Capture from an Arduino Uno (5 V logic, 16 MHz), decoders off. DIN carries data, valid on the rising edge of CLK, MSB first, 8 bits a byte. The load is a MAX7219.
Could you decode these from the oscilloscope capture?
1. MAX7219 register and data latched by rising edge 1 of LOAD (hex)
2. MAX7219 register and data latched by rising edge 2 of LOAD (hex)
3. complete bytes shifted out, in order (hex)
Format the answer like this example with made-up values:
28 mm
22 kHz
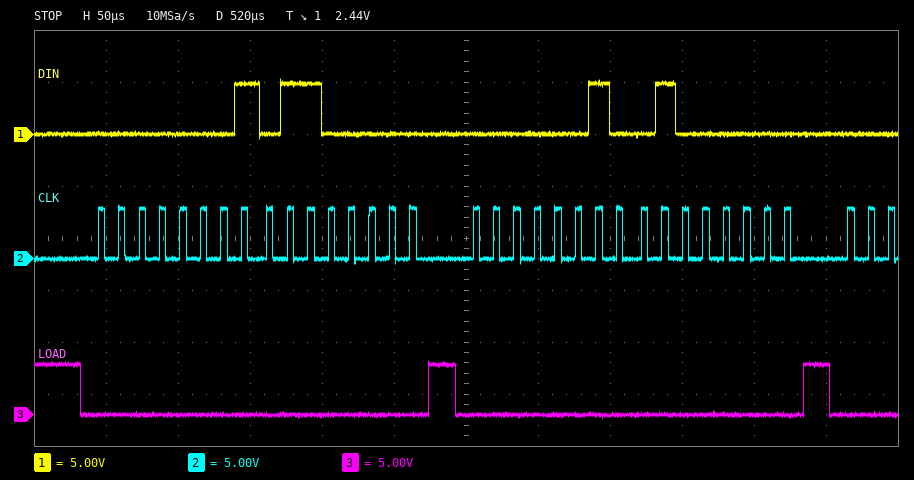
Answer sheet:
register 0x1, data 0x60
register 0x2, data 0x40
0x01 0x60 0x02 0x40
